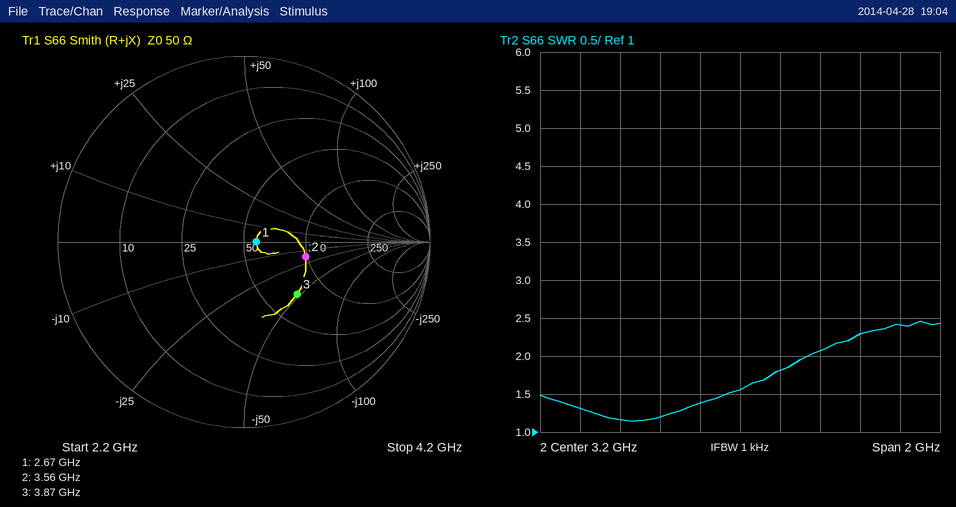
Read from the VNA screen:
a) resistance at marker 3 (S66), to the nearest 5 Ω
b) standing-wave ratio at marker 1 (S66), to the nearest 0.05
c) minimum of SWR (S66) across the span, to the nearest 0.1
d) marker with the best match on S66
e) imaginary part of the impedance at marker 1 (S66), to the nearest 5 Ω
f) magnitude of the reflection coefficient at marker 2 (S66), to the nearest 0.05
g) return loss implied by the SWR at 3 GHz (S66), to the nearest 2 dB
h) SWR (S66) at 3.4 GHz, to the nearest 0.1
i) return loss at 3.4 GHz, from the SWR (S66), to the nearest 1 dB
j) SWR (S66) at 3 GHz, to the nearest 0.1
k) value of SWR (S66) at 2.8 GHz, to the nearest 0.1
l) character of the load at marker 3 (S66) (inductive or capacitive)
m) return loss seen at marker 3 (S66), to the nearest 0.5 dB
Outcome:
70 Ω
1.15
1.1
marker 1
0 Ω
0.35
16 dB
1.8
11 dB
1.4
1.2
capacitive
8.0 dB
